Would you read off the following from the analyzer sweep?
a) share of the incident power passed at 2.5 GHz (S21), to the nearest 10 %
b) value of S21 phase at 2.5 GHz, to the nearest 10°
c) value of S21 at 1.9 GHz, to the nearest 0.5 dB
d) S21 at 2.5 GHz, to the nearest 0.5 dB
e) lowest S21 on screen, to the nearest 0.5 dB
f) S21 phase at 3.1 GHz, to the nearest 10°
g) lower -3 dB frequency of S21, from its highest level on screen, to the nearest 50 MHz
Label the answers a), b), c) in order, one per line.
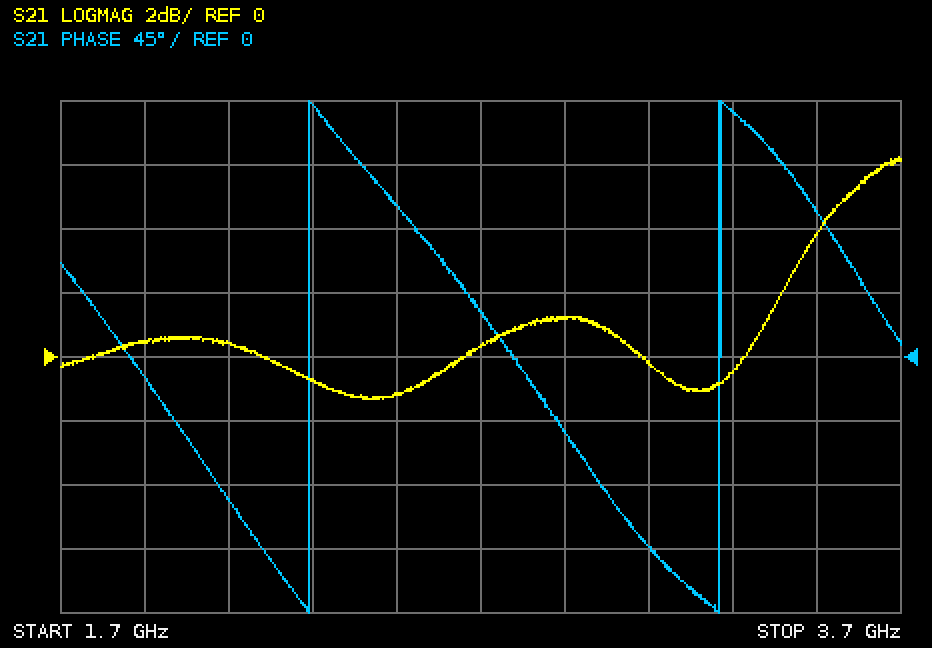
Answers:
a) 80 %
b) 110°
c) 0.5 dB
d) -1.0 dB
e) -1.5 dB
f) -130°
g) 3.45 GHz
